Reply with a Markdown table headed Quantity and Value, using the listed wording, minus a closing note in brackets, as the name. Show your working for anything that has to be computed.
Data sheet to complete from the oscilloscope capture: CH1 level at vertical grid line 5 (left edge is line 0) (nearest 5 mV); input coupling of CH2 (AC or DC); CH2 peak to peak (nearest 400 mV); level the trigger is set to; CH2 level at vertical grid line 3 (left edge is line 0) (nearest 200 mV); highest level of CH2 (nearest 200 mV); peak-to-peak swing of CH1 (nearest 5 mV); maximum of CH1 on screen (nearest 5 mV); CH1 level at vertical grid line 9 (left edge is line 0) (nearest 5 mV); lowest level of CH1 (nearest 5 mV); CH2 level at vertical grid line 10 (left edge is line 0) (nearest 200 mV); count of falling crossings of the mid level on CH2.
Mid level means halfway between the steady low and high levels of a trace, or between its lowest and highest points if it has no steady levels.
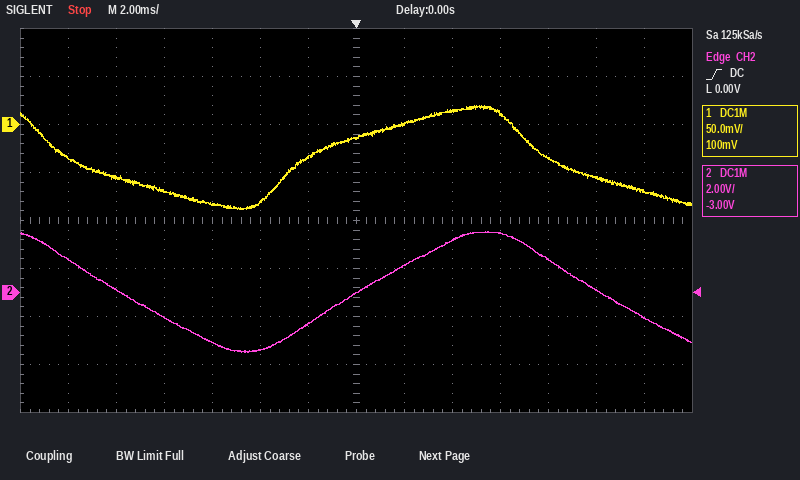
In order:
| Quantity | Value |
|---|---|
| CH1 level at vertical grid line 5 (left edge is line 0) | -80 mV |
| input coupling of CH2 | DC |
| CH2 peak to peak | 5.2 V |
| level the trigger is set to | 0.00 V |
| CH2 level at vertical grid line 3 (left edge is line 0) | -1.0 V |
| highest level of CH2 | 2.6 V |
| peak-to-peak swing of CH1 | 20 mV − (-90 mV) = 110 mV |
| maximum of CH1 on screen | 20 mV |
| CH1 level at vertical grid line 9 (left edge is line 0) | 15 mV |
| lowest level of CH1 | -90 mV |
| CH2 level at vertical grid line 10 (left edge is line 0) | 2.4 V |
| count of falling crossings of the mid level on CH2 | 2 |
